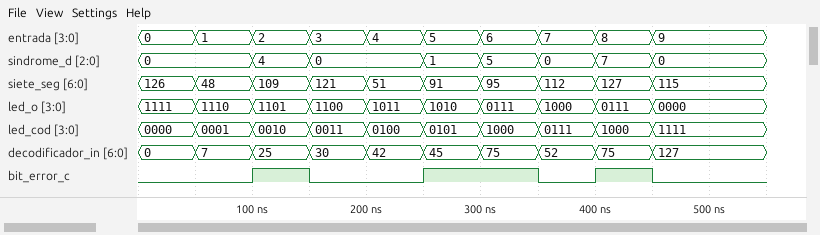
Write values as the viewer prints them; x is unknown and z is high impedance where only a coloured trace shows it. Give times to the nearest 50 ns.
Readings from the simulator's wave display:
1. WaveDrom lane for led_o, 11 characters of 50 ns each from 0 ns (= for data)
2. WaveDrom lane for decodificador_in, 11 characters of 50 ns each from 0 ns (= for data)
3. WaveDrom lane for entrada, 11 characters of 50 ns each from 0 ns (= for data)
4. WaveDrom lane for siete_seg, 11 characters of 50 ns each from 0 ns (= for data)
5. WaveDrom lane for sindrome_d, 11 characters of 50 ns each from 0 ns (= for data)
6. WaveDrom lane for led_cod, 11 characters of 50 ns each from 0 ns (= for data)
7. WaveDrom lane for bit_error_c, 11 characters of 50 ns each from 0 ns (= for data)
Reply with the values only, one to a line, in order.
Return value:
{name: 'led_o', wave: '==========.', data: '1111 1110 1101 1100 1011 1010 0111 1000 0111 0000'}
{name: 'decodificador_in', wave: '==========.', data: '0 7 25 30 42 45 75 52 75 127'}
{name: 'entrada', wave: '==========.', data: '0 1 2 3 4 5 6 7 8 9'}
{name: 'siete_seg', wave: '==========.', data: '126 48 109 121 51 91 95 112 127 115'}
{name: 'sindrome_d', wave: '=.==.=====.', data: '0 4 0 1 5 0 7 0'}
{name: 'led_cod', wave: '==========.', data: '0000 0001 0010 0011 0100 0101 1000 0111 1000 1111'}
{name: 'bit_error_c', wave: '0.10.1.010.'}
